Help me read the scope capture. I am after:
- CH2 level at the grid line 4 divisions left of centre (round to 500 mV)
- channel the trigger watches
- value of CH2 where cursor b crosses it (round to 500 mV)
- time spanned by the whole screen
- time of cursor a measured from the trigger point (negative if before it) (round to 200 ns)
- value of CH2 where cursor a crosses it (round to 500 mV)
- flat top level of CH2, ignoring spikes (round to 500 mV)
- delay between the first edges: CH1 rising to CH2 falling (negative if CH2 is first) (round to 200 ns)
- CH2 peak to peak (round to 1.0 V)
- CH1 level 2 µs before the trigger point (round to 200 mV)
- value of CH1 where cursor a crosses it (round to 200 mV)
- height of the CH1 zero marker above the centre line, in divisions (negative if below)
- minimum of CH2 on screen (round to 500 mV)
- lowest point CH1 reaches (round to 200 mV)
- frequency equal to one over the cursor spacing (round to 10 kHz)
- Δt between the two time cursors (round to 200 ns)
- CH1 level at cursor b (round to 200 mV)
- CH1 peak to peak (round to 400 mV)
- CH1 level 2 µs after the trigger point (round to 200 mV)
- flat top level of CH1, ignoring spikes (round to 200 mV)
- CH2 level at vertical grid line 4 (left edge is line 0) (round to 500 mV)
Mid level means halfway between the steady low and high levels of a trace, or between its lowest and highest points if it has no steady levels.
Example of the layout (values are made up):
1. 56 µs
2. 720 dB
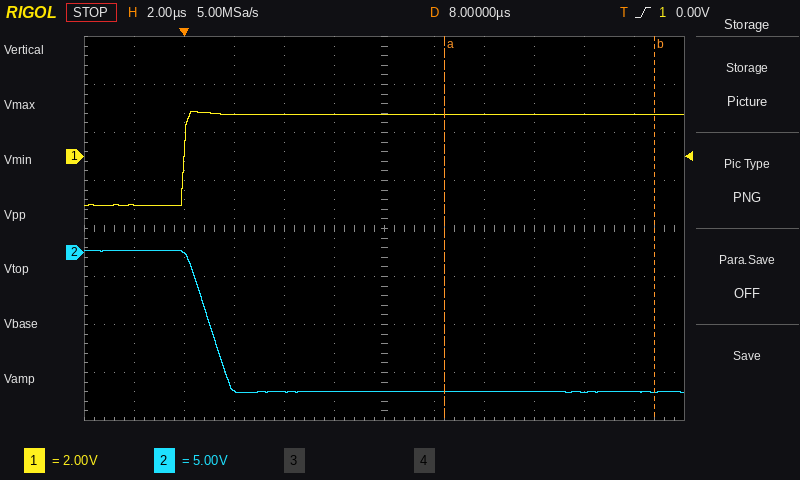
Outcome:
1. 0.0 V
2. CH1
3. -14.5 V
4. 24 µs
5. +10.4 µs
6. -14.5 V
7. 0.0 V
8. +1.0 µs
9. 15.0 V
10. -2.0 V
11. 1.8 V
12. +1.5 div
13. -14.5 V
14. -2.0 V
15. 120 kHz
16. 8.4 µs
17. 1.8 V
18. 4.0 V
19. 1.8 V
20. 1.8 V
21. -14.5 V
